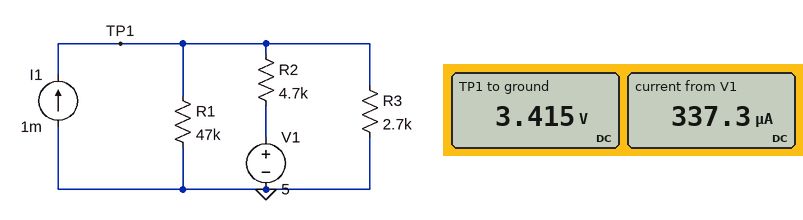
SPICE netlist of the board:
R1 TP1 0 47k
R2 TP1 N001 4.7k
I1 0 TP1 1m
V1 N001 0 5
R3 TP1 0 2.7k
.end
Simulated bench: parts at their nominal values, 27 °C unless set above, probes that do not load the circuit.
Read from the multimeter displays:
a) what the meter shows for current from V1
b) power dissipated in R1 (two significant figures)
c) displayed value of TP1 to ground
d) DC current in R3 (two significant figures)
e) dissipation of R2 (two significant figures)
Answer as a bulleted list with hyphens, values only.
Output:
- 337.3 µA
- 250 µW
- 3.415 V
- 1.3 mA
- 530 µW
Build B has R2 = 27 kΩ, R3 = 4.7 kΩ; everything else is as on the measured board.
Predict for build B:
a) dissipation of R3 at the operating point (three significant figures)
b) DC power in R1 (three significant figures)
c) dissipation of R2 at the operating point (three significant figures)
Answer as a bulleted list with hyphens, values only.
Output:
- 4.07 mW
- 407 µW
- 14.6 µW
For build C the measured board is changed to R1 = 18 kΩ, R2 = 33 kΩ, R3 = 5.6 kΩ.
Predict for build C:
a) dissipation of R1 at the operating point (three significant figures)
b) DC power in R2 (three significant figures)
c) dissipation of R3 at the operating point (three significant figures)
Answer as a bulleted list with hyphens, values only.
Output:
- 1.05 mW
- 12.6 µW
- 3.39 mW
